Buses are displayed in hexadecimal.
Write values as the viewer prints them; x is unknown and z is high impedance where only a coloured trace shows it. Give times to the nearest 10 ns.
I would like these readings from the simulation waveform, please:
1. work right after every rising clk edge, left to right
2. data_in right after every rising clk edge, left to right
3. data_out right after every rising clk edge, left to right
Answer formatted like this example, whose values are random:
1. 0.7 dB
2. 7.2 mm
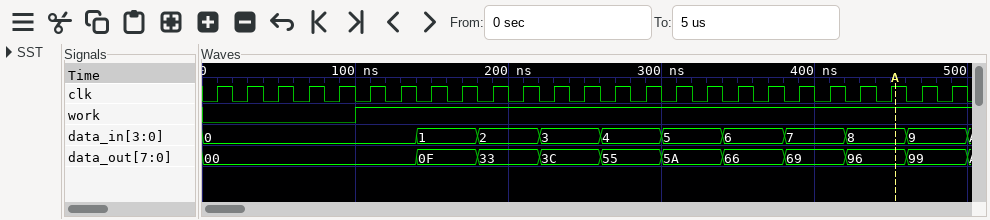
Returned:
1. 0 0 0 0 0 1 1 1 1 1 1 1 1 1 1 1 1 1 1 1 1 1 1 1 1
2. 0, 0, 0, 0, 0, 0, 0, 1, 1, 2, 2, 3, 3, 4, 4, 5, 5, 6, 6, 7, 7, 8, 8, 9, 9
3. 00, 00, 00, 00, 00, 00, 00, 0F, 0F, 33, 33, 3C, 3C, 55, 55, 5A, 5A, 66, 66, 69, 69, 96, 96, 99, 99
